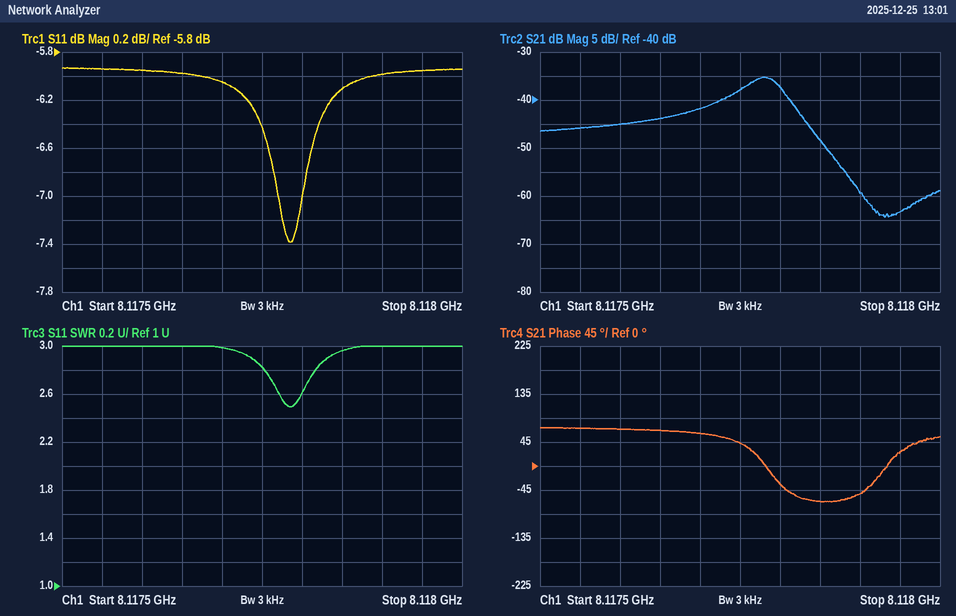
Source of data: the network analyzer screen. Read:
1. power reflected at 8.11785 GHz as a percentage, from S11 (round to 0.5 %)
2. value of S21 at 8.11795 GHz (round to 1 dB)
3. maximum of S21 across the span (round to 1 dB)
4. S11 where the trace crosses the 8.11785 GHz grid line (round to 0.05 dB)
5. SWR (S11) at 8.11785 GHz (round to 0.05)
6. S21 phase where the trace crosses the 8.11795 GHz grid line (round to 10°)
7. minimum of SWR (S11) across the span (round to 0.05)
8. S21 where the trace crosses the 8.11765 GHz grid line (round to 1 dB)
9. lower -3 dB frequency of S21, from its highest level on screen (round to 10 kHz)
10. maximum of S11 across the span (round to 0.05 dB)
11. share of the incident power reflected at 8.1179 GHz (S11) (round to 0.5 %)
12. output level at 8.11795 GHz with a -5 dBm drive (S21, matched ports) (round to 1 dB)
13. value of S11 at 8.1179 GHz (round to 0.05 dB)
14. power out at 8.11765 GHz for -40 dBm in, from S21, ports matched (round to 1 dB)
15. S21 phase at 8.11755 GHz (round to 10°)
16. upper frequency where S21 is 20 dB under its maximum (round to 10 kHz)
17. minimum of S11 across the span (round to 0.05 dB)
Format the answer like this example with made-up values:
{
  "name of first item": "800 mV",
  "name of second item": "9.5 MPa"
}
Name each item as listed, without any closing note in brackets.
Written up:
{
  "power reflected at 8.11785 GHz as a percentage, from S11": "24.5 %",
  "value of S21 at 8.11795 GHz": "-63 dB",
  "maximum of S21 across the span": "-35 dB",
  "S11 where the trace crosses the 8.11785 GHz grid line": "-6.10 dB",
  "SWR (S11) at 8.11785 GHz": "2.95",
  "S21 phase where the trace crosses the 8.11795 GHz grid line": "30°",
  "minimum of SWR (S11) across the span": "2.50",
  "S21 where the trace crosses the 8.11765 GHz grid line": "-44 dB",
  "lower -3 dB frequency of S21, from its highest level on screen": "8.11775 GHz",
  "maximum of S11 across the span": "-5.95 dB",
  "share of the incident power reflected at 8.1179 GHz (S11)": "25.0 %",
  "output level at 8.11795 GHz with a -5 dBm drive (S21, matched ports)": "-68 dBm",
  "value of S11 at 8.1179 GHz": "-6.00 dB",
  "power out at 8.11765 GHz for -40 dBm in, from S21, ports matched": "-84 dBm",
  "S21 phase at 8.11755 GHz": "70°",
  "upper frequency where S21 is 20 dB under its maximum": "8.11788 GHz",
  "minimum of S11 across the span": "-7.40 dB"
}
